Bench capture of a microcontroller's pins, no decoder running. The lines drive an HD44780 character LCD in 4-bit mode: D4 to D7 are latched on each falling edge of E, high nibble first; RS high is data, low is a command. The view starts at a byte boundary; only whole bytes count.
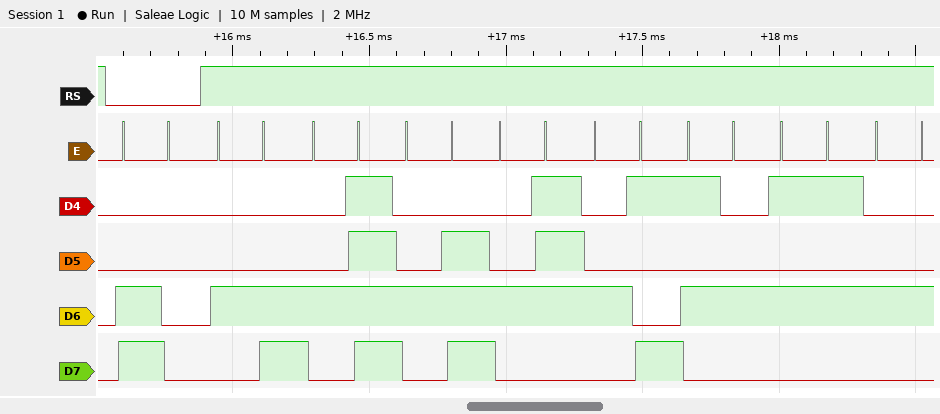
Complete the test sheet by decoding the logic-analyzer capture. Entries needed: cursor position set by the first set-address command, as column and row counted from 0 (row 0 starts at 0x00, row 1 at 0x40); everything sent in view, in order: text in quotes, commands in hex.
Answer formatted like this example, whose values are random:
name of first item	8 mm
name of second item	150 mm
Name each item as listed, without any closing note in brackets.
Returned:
cursor position set by the first set-address command, as column and row counted from 0	column 0, row 1
everything sent in view, in order: text in quotes, commands in hex	0xC0 "LONGITUD"
